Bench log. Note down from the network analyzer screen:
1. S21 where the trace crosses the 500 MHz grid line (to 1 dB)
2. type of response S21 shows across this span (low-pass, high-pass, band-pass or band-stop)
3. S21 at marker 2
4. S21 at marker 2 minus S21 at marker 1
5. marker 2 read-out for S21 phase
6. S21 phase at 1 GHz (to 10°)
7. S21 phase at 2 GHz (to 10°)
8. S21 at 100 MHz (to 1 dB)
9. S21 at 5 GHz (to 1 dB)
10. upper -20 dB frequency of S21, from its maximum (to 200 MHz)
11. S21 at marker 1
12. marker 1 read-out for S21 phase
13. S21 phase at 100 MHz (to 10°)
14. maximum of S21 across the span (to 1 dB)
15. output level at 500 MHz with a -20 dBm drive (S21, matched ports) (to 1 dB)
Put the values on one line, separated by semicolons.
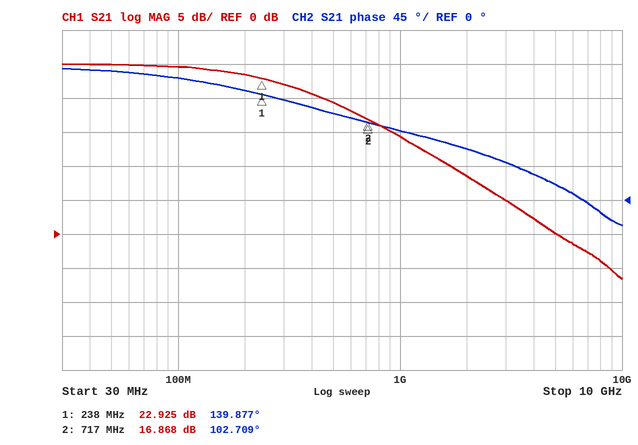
19 dB; low-pass; 16.868 dB; -6.057 dB; 102.709°; 90°; 70°; 25 dB; 0 dB; 3.0 GHz; 22.925 dB; 139.877°; 160°; 25 dB; -1 dBm
